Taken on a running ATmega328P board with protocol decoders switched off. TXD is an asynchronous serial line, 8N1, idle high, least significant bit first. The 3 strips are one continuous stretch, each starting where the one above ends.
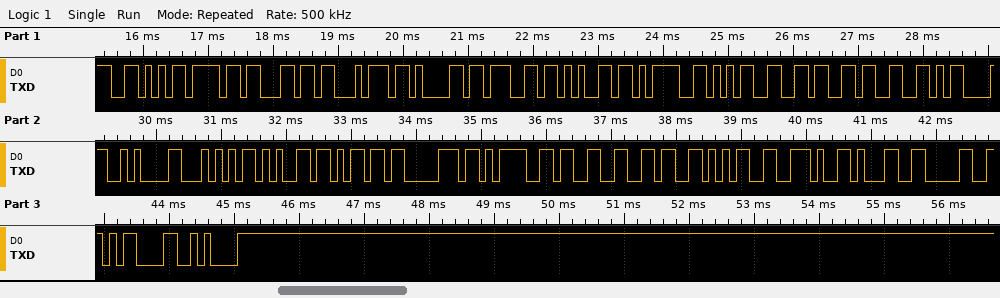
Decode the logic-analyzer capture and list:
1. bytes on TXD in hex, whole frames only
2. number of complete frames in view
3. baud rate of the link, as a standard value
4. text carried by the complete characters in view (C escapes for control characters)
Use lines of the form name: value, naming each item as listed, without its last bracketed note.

bytes on TXD in hex, whole frames only: 56 6F 6C 74 61 67 65 3D 35 36 33 0D 0A 54 65 6D 70 3D 33 36 35 2E 31 30 0D 0A
number of complete frames in view: 26
baud rate of the link, as a standard value: 9600 baud
text carried by the complete characters in view: "Voltage=563\r\nTemp=365.10\r\n"
